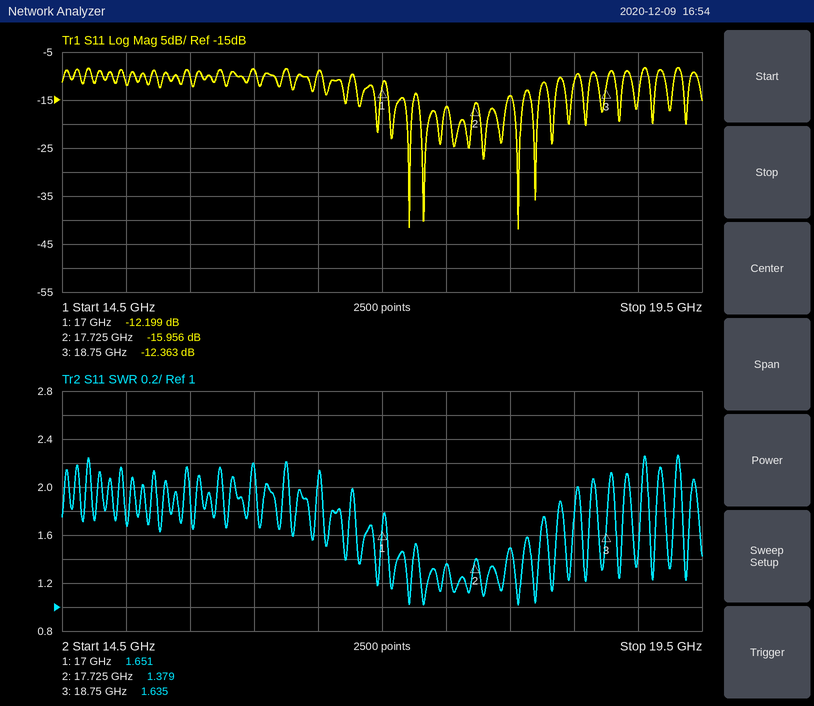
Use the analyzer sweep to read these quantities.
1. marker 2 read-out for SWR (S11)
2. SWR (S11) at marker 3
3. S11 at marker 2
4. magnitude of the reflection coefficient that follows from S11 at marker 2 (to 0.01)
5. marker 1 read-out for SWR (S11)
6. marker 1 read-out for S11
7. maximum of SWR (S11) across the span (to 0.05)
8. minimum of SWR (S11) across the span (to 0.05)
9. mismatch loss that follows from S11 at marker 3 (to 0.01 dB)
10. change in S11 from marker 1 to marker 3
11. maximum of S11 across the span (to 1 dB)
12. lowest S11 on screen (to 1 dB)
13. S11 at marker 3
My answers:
1.379
1.635
-15.956 dB
0.16
1.651
-12.199 dB
2.25
1.00
0.26 dB
-0.164 dB
-8 dB
-42 dB
-12.363 dB
